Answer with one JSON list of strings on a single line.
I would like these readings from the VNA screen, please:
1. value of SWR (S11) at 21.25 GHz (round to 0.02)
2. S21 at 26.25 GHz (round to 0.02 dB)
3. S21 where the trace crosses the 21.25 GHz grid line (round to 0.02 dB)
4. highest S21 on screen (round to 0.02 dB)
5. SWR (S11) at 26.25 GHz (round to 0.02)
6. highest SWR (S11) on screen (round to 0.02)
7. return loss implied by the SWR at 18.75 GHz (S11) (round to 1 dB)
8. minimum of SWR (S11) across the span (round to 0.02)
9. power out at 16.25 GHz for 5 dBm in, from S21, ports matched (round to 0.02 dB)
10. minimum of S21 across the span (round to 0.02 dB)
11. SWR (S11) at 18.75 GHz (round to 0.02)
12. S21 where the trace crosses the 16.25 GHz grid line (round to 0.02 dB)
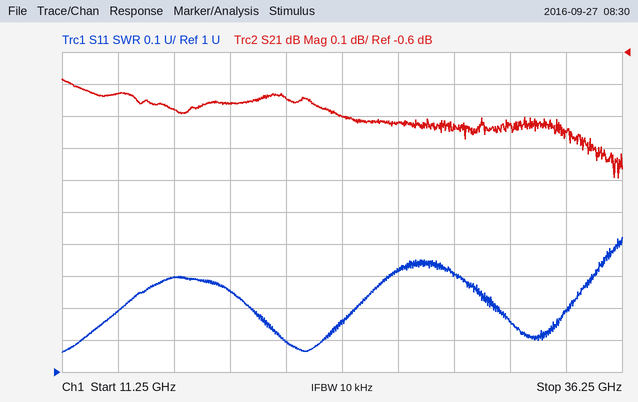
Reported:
["1.10", "-0.82 dB", "-0.74 dB", "-0.68 dB", "1.32", "1.42", "19 dB", "1.06", "4.22 dBm", "-1.00 dB", "1.26", "-0.78 dB"]
